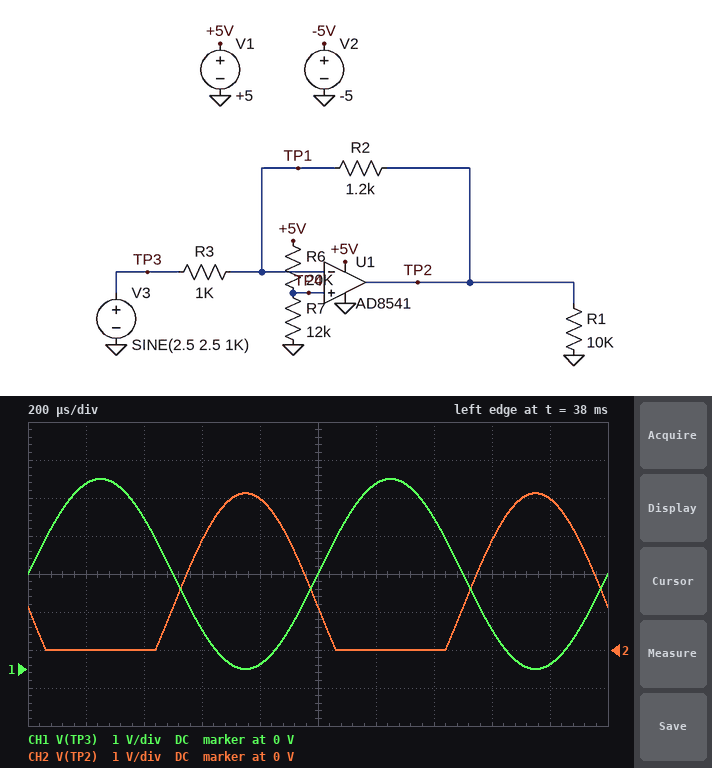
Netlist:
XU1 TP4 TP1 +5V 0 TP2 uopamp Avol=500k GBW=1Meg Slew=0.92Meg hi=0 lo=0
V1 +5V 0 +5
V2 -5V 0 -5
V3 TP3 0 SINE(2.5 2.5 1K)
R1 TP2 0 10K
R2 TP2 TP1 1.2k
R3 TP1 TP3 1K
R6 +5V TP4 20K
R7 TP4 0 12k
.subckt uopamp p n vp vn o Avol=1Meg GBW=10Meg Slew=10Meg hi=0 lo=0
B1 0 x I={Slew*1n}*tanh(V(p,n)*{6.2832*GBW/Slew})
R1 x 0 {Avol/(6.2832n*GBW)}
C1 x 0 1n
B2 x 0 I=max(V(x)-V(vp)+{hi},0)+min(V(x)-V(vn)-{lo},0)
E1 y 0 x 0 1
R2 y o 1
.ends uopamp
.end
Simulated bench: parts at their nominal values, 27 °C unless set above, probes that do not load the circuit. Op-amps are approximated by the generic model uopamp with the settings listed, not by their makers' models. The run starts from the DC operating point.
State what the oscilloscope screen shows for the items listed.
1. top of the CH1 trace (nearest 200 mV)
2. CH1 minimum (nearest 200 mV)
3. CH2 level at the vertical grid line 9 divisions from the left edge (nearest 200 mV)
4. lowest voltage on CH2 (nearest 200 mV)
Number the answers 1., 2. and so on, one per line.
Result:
1. 5.0 V
2. 0 V
3. 4.0 V
4. 0 V
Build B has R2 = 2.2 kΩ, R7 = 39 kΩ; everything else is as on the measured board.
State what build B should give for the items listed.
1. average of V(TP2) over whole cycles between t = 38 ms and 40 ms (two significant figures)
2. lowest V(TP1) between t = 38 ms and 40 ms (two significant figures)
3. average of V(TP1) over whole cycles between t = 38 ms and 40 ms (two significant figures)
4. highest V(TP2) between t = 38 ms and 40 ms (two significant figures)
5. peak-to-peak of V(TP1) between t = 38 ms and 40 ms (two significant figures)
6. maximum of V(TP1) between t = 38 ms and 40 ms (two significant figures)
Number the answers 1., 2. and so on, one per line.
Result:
1. 3.3 V
2. 1.6 V
3. 2.8 V
4. 5.0 V
5. 1.9 V
6. 3.4 V
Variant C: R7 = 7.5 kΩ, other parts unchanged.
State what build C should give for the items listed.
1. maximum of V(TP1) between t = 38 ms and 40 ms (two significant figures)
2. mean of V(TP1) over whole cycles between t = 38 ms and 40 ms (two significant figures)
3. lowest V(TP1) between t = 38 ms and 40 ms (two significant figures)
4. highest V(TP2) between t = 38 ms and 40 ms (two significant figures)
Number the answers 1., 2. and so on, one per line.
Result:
1. 2.7 V
2. 1.8 V
3. 1.4 V
4. 3.0 V
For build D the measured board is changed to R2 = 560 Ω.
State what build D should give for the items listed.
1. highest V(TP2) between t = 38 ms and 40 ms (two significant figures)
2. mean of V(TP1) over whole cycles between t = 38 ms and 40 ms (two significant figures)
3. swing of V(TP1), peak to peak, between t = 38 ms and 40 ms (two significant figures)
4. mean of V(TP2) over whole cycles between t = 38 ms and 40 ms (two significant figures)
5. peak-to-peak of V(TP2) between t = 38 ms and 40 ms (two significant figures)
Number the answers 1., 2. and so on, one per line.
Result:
1. 2.9 V
2. 1.9 V
3. 2.8 mV
4. 1.5 V
5. 2.8 V
